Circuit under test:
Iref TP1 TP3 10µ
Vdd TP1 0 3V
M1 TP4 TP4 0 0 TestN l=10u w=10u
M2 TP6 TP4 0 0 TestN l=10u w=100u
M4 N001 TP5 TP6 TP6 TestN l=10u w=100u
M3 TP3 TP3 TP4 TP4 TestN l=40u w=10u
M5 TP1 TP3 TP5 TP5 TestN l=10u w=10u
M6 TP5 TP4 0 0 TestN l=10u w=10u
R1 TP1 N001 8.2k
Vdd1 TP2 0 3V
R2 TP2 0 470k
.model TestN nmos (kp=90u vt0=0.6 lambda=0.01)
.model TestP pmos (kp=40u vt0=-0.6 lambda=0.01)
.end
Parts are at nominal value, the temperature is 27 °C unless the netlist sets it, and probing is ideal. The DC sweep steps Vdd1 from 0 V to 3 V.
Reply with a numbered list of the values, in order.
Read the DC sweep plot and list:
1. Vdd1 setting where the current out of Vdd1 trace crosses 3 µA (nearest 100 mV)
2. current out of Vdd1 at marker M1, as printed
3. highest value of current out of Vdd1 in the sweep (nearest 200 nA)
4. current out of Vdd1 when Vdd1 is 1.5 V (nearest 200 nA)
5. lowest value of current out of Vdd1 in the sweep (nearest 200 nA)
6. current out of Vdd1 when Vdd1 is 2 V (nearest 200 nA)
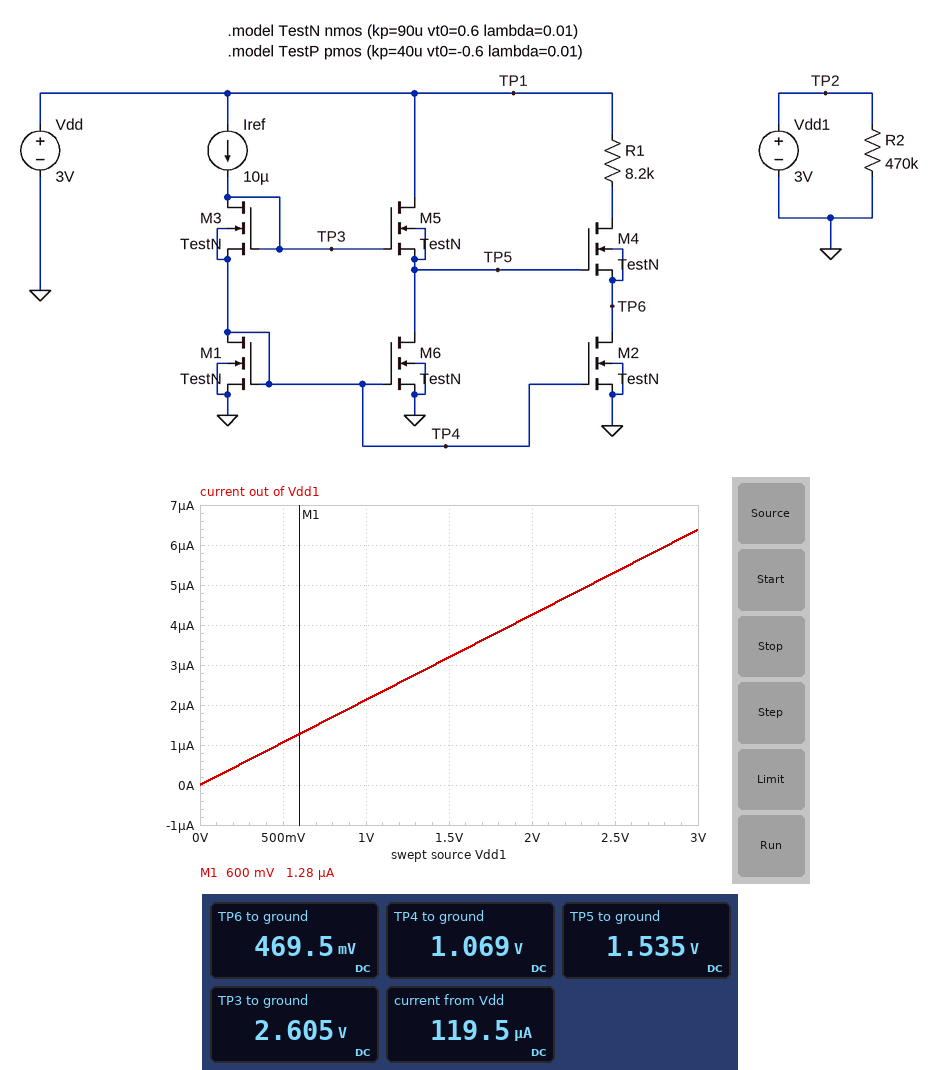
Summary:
1. 1.4 V
2. 1.28 µA
3. 6.4 µA
4. 3.2 µA
5. 0 A
6. 4.2 µA
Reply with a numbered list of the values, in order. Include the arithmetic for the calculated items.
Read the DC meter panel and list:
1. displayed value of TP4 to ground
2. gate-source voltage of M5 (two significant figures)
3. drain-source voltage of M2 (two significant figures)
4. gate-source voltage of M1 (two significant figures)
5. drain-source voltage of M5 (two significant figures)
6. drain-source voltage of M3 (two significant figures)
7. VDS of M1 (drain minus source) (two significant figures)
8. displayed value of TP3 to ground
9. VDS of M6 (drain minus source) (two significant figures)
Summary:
1. 1.069 V
2. 2.605 V - 1.535 V = 1.1 V
3. 469.5 mV = 470 mV
4. 1.069 V = 1.1 V
5. 3 V - 1.535 V = 1.5 V
6. 2.605 V - 1.069 V = 1.5 V
7. 1.069 V = 1.1 V
8. 2.605 V
9. 1.535 V = 1.5 V
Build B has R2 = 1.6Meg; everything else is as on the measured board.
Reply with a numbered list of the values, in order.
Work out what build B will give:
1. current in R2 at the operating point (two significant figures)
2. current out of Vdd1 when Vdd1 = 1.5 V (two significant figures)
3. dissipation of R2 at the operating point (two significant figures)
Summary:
1. 1.9 µA
2. 940 nA
3. 5.6 µW
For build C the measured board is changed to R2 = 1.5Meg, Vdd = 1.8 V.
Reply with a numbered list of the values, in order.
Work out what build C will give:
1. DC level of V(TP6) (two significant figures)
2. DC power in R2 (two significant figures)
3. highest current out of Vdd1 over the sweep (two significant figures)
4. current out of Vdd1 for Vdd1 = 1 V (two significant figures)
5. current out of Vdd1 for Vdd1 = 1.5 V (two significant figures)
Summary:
1. 420 mV
2. 6.0 µW
3. 2.0 µA
4. 670 nA
5. 1.0 µA
